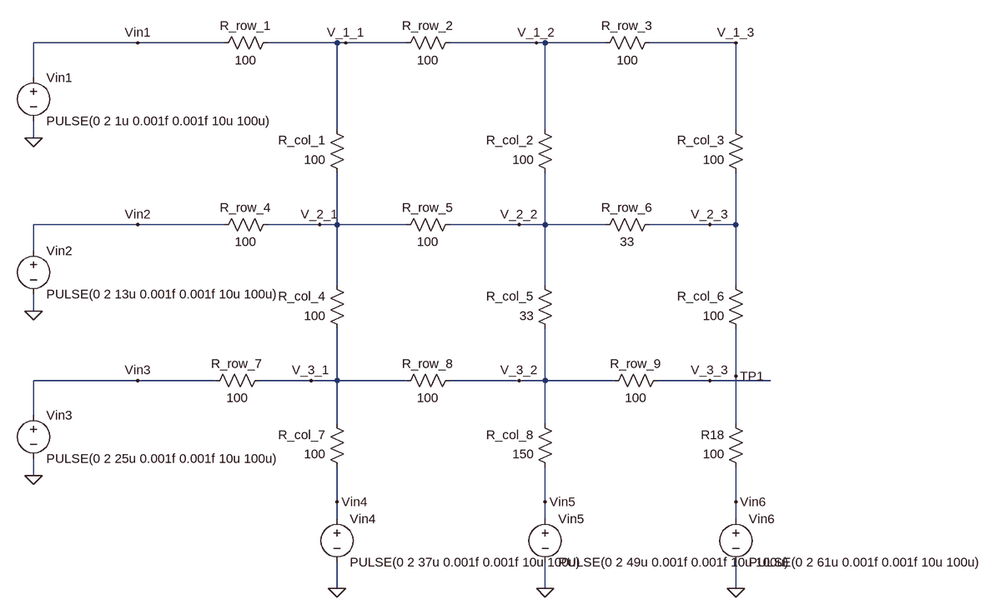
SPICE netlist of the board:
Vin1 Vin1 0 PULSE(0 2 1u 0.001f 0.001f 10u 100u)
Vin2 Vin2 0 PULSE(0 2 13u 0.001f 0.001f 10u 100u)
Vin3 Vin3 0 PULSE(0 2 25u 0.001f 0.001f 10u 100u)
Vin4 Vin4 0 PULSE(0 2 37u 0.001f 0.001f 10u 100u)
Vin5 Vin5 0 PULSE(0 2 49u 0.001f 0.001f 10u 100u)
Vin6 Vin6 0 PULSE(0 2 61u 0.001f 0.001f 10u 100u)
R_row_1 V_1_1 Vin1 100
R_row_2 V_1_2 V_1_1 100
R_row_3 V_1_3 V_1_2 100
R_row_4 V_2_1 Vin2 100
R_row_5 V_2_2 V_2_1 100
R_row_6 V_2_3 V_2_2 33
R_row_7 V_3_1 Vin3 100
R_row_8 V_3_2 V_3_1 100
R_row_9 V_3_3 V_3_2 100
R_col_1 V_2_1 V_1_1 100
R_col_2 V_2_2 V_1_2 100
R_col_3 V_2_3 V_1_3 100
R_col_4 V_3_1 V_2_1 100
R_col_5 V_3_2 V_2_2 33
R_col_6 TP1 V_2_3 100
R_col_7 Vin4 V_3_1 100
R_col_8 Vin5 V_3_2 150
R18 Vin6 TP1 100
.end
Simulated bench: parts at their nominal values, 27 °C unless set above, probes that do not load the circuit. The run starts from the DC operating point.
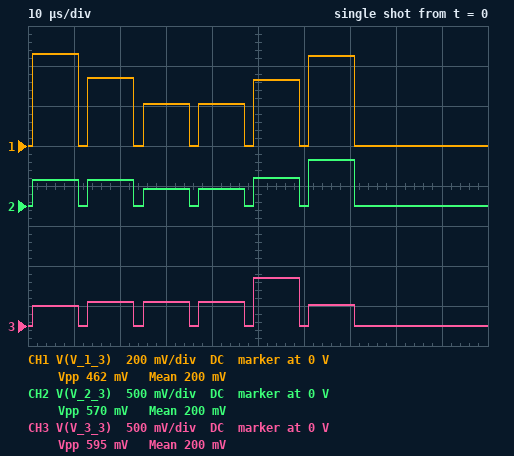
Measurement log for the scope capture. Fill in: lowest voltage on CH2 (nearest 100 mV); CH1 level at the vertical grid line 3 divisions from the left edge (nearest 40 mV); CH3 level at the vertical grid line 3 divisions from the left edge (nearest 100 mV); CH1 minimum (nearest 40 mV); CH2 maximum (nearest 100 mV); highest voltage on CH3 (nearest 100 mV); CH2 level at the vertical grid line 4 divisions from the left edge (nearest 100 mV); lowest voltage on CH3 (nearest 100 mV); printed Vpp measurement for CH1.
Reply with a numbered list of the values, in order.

1. 0 V
2. 200 mV
3. 300 mV
4. 0 V
5. 600 mV
6. 600 mV
7. 200 mV
8. 0 V
9. 462 mV
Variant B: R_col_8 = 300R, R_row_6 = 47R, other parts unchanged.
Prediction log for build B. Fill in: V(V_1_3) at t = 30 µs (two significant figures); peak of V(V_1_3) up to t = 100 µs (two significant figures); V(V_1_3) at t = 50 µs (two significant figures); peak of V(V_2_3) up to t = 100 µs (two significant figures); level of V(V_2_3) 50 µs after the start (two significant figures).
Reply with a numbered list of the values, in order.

1. 230 mV
2. 500 mV
3. 190 mV
4. 640 mV
5. 200 mV
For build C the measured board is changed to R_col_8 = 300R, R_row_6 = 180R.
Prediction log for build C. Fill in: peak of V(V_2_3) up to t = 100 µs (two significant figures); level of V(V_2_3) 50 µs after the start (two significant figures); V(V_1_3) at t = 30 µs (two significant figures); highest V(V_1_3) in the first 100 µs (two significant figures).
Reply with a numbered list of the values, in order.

1. 870 mV
2. 150 mV
3. 210 mV
4. 610 mV
